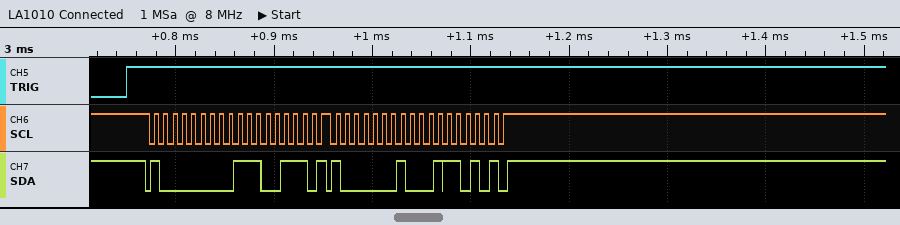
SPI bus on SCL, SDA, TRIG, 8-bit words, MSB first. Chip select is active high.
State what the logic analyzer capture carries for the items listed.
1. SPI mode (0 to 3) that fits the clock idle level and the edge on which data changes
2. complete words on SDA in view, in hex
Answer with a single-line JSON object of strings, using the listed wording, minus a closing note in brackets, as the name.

{"SPI mode (0 to 3) that fits the clock idle level and the edge on which data changes": "3", "complete words on SDA in view, in hex": "80, 73, B0, 23"}
